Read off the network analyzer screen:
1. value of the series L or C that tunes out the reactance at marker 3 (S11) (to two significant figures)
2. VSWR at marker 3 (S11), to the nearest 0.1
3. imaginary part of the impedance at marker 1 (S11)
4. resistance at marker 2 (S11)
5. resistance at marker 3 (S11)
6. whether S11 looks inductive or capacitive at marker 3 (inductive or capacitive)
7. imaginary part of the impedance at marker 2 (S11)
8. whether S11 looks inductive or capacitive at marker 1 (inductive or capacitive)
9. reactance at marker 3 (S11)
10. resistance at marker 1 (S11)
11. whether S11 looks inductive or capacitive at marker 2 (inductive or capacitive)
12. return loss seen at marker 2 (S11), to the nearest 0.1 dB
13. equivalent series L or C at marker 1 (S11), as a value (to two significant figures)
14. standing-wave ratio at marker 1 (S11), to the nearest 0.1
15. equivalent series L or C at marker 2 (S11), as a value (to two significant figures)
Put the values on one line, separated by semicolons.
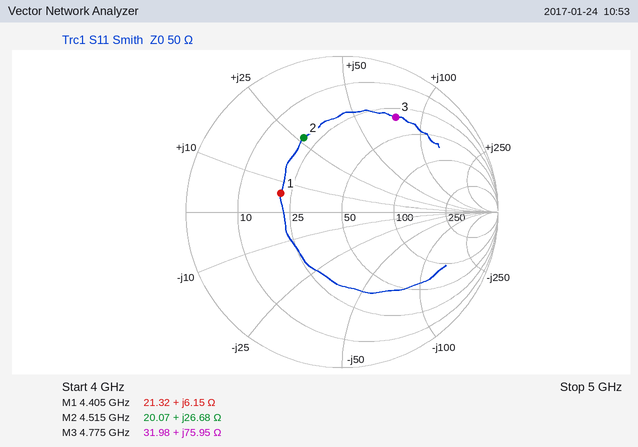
440 fF; 5.6; +6.15 Ω; 20.07 Ω; 31.98 Ω; inductive; +26.68 Ω; inductive; +75.95 Ω; 21.32 Ω; inductive; 5.4 dB; 220 pH; 2.4; 940 pH
